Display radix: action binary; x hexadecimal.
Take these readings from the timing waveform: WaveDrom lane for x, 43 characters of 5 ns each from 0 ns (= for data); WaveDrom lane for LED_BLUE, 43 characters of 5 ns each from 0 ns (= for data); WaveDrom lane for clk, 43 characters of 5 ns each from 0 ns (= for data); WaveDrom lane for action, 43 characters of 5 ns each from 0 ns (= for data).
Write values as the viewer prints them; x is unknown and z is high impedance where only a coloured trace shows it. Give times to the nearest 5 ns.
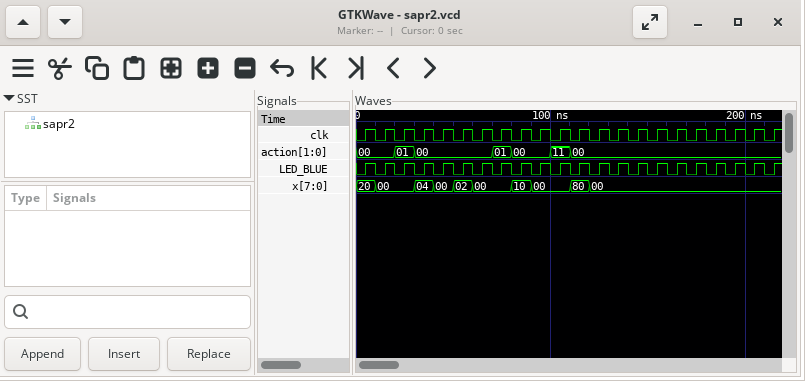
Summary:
{name: 'x', wave: '=.=...=.=.=.=...=.=...=.=..................', data: '20 00 04 00 02 00 10 00 80 00'}
{name: 'LED_BLUE', wave: '0101010101010101010101010101010101010101010'}
{name: 'clk', wave: '0101010101010101010101010101010101010101010'}
{name: 'action', wave: '=...=.=.......=.=...=.=....................', data: '00 01 00 01 00 11 00'}
